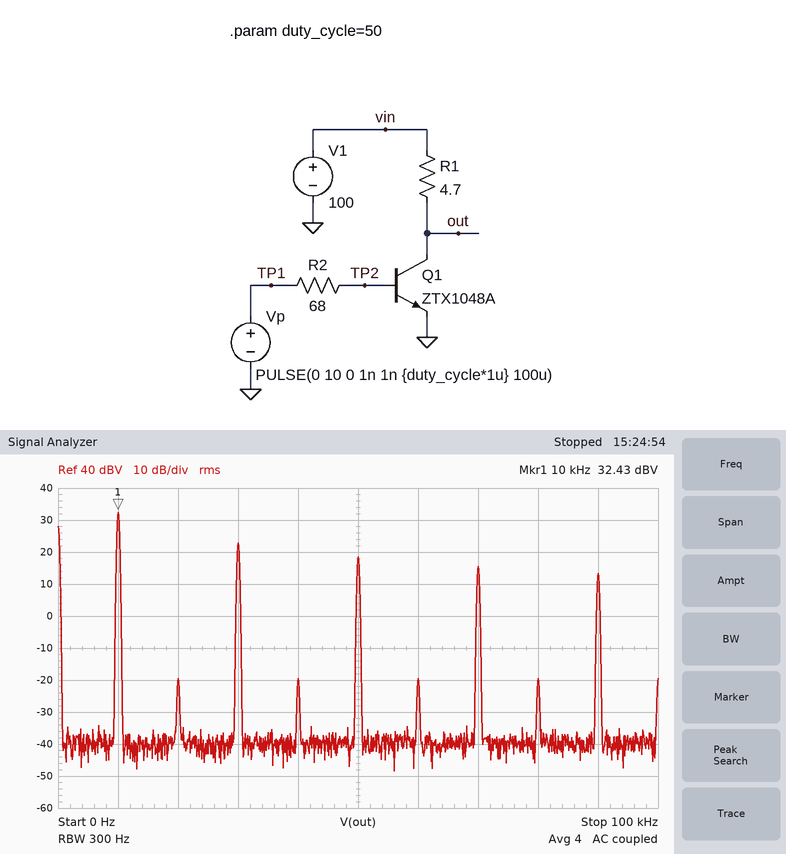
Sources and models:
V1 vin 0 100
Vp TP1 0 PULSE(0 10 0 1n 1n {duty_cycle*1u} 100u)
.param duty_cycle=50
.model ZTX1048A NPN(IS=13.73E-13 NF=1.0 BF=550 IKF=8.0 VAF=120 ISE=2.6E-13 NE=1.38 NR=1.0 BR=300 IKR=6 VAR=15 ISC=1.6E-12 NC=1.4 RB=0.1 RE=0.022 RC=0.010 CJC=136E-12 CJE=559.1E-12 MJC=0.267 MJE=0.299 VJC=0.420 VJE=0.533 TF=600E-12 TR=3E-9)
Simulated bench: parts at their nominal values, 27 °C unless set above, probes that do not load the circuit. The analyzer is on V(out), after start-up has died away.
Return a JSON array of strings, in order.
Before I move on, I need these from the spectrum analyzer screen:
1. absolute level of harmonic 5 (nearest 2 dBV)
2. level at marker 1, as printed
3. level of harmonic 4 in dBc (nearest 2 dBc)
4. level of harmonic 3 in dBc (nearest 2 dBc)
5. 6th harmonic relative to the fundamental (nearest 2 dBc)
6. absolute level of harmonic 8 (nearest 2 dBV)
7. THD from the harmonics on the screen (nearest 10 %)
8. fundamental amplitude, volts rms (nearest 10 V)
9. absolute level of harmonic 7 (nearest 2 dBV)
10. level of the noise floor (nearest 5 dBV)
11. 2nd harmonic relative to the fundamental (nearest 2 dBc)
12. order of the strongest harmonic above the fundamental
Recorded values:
["18 dBV", "32.43 dBV", "-52 dBc", "-10 dBc", "-52 dBc", "-20 dBV", "40 %", "40 V", "16 dBV", "-40 dBV", "-52 dBc", "3"]
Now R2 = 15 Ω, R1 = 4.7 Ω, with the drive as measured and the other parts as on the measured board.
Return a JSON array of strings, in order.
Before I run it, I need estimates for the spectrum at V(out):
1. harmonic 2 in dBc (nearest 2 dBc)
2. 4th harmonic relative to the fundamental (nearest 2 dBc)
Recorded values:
["-36 dBc", "-36 dBc"]
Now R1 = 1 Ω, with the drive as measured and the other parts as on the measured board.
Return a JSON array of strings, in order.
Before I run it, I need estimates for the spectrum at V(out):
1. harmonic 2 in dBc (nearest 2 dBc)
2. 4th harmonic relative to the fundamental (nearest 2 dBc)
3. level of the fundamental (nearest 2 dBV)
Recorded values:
["-56 dBc", "-56 dBc", "22 dBV"]
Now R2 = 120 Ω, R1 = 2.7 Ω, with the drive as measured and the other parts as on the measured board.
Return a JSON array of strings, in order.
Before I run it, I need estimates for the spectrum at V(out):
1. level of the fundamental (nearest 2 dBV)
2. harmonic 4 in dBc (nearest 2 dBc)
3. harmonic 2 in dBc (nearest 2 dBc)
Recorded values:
["28 dBV", "-54 dBc", "-54 dBc"]
